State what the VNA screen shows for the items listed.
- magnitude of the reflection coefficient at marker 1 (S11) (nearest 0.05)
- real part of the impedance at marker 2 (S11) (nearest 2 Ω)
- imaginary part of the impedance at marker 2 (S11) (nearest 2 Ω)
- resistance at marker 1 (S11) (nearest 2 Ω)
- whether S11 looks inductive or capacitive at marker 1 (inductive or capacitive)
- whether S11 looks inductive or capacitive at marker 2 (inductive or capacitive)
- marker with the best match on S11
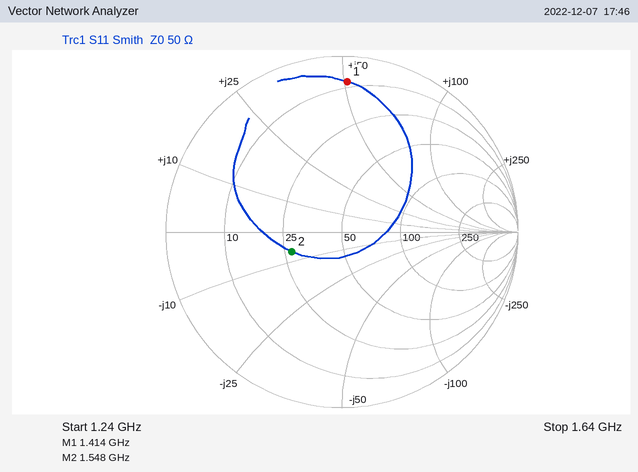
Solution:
0.85
28 Ω
-6 Ω
8 Ω
inductive
capacitive
marker 2
